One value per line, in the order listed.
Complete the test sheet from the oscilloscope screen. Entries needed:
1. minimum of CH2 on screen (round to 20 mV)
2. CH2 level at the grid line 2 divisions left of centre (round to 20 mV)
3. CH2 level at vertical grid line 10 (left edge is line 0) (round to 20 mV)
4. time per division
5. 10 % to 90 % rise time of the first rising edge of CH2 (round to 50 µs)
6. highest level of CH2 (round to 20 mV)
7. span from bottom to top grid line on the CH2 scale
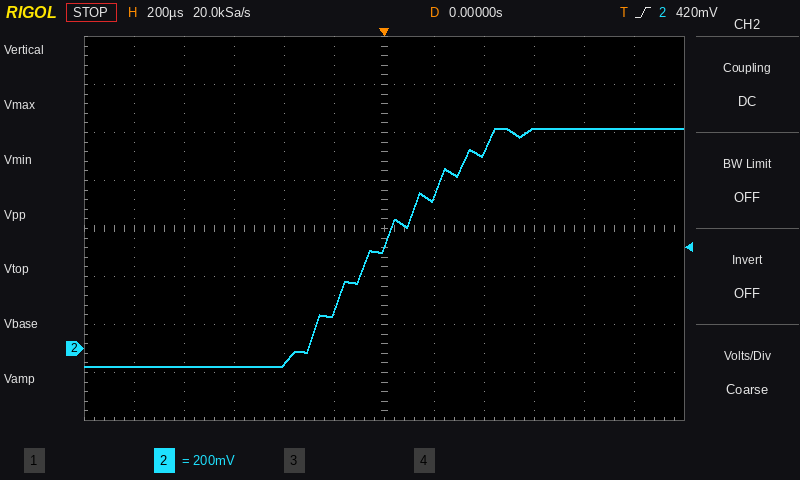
-80 mV
-60 mV
920 mV
200 µs
650 µs
920 mV
1.6 V
